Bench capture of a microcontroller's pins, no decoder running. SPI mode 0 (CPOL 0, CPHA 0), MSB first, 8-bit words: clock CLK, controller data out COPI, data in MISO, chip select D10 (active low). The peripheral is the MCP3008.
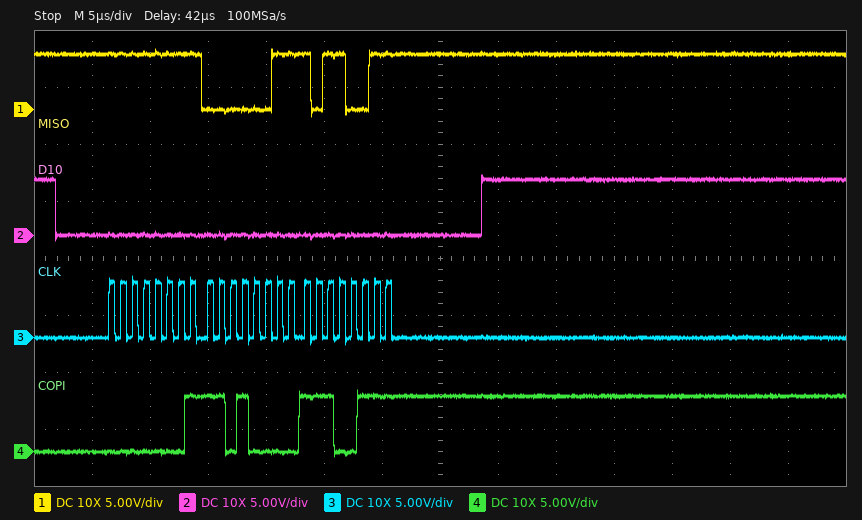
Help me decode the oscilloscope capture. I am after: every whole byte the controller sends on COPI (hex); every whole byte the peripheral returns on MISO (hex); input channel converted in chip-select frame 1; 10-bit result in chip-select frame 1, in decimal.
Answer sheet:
01 D0 E7
FF 03 B3
5
947
